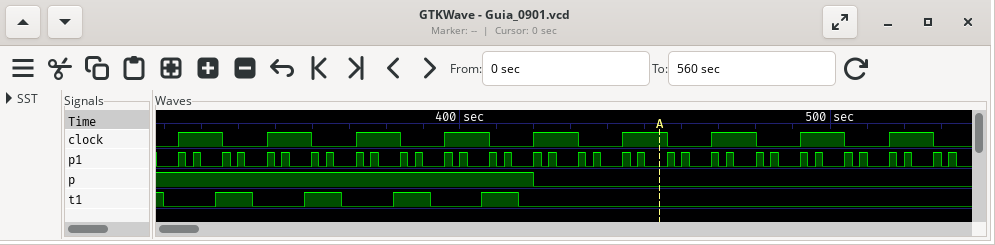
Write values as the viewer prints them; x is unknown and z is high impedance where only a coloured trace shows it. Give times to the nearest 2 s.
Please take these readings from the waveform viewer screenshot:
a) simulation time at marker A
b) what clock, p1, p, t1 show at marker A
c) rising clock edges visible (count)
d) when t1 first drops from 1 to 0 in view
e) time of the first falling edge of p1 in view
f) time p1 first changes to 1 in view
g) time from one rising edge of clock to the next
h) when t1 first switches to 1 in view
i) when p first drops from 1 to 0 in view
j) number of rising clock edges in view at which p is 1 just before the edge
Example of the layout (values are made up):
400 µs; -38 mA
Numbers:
454 s; clock=1, p1=0, p=0, t1=0; 9; 320 s; 326 s; 324 s; 24 s; 334 s; 420 s; 5
